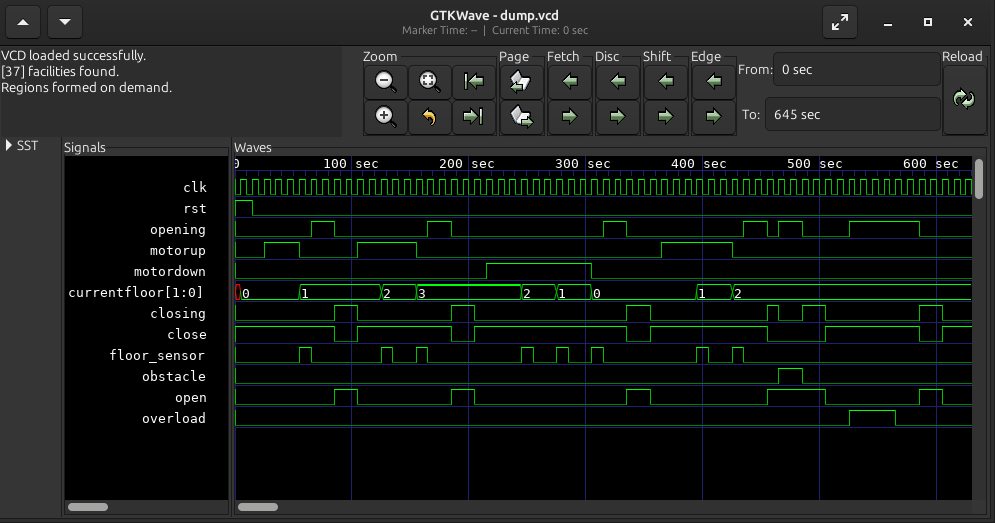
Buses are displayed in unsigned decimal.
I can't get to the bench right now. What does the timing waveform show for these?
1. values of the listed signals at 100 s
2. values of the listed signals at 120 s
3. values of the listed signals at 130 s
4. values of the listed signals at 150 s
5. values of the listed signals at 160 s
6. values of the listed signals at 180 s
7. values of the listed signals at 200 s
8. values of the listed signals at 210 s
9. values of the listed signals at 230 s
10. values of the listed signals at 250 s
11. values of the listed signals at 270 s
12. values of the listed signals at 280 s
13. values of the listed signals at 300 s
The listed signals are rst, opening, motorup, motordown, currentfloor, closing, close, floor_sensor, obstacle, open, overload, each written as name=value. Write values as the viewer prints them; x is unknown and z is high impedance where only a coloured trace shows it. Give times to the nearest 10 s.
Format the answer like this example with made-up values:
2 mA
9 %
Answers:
rst=0, opening=0, motorup=0, motordown=0, currentfloor=1, closing=1, close=0, floor_sensor=0, obstacle=0, open=1, overload=0
rst=0, opening=0, motorup=1, motordown=0, currentfloor=1, closing=0, close=1, floor_sensor=0, obstacle=0, open=0, overload=0
rst=0, opening=0, motorup=1, motordown=0, currentfloor=2, closing=0, close=1, floor_sensor=1, obstacle=0, open=0, overload=0
rst=0, opening=0, motorup=1, motordown=0, currentfloor=2, closing=0, close=1, floor_sensor=0, obstacle=0, open=0, overload=0
rst=0, opening=0, motorup=0, motordown=0, currentfloor=3, closing=0, close=1, floor_sensor=1, obstacle=0, open=0, overload=0
rst=0, opening=1, motorup=0, motordown=0, currentfloor=3, closing=0, close=1, floor_sensor=0, obstacle=0, open=0, overload=0
rst=0, opening=0, motorup=0, motordown=0, currentfloor=3, closing=1, close=0, floor_sensor=0, obstacle=0, open=1, overload=0
rst=0, opening=0, motorup=0, motordown=0, currentfloor=3, closing=0, close=1, floor_sensor=0, obstacle=0, open=0, overload=0
rst=0, opening=0, motorup=0, motordown=1, currentfloor=3, closing=0, close=1, floor_sensor=0, obstacle=0, open=0, overload=0
rst=0, opening=0, motorup=0, motordown=1, currentfloor=2, closing=0, close=1, floor_sensor=1, obstacle=0, open=0, overload=0
rst=0, opening=0, motorup=0, motordown=1, currentfloor=2, closing=0, close=1, floor_sensor=0, obstacle=0, open=0, overload=0
rst=0, opening=0, motorup=0, motordown=1, currentfloor=1, closing=0, close=1, floor_sensor=1, obstacle=0, open=0, overload=0
rst=0, opening=0, motorup=0, motordown=1, currentfloor=1, closing=0, close=1, floor_sensor=0, obstacle=0, open=0, overload=0
